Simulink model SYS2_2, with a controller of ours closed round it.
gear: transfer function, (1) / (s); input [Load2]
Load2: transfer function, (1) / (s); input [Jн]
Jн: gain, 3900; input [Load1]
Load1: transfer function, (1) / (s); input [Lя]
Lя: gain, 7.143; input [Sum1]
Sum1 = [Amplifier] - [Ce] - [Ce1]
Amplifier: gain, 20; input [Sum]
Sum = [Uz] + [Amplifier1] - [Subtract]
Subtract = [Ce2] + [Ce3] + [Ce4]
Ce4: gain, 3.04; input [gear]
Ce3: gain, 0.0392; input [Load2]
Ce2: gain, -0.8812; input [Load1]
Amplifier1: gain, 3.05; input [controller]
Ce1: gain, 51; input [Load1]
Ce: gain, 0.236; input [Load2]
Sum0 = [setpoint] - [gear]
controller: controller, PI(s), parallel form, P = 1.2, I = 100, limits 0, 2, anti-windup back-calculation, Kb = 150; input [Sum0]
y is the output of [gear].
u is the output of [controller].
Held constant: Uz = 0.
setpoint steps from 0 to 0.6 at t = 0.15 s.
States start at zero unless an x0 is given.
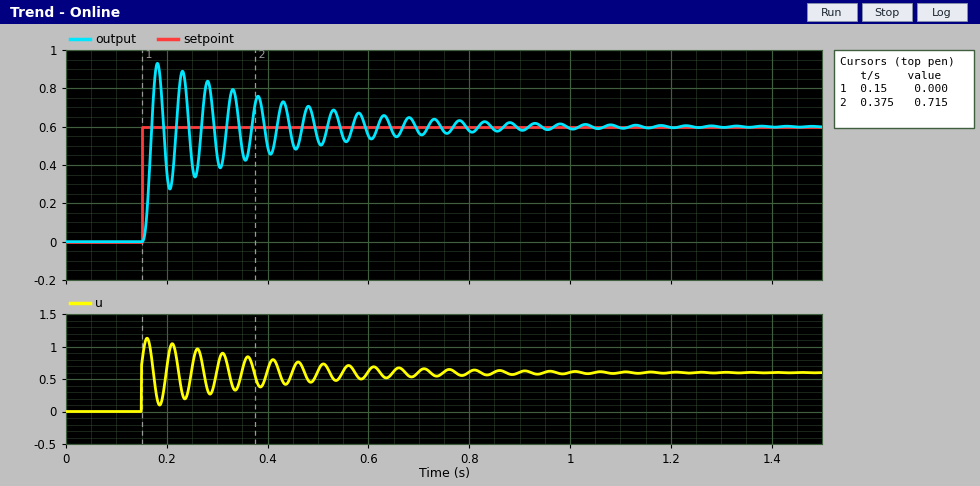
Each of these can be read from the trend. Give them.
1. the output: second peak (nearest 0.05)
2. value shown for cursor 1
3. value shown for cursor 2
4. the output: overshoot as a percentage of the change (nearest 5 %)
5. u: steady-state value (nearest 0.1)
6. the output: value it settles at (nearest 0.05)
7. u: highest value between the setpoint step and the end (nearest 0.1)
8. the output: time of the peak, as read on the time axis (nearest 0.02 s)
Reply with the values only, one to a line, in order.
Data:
0.90
0.000
0.715
55 %
0.6
0.60
1.1
0.18 s
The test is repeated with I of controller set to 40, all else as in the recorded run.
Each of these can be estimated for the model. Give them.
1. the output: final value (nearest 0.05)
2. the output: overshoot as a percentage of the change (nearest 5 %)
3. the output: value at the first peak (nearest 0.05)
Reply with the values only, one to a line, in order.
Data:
0.60
10 %
0.65
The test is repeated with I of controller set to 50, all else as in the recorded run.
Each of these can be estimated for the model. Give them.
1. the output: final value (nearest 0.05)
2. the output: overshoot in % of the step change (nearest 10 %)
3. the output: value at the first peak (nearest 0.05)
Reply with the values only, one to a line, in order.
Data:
0.60
20 %
0.70
